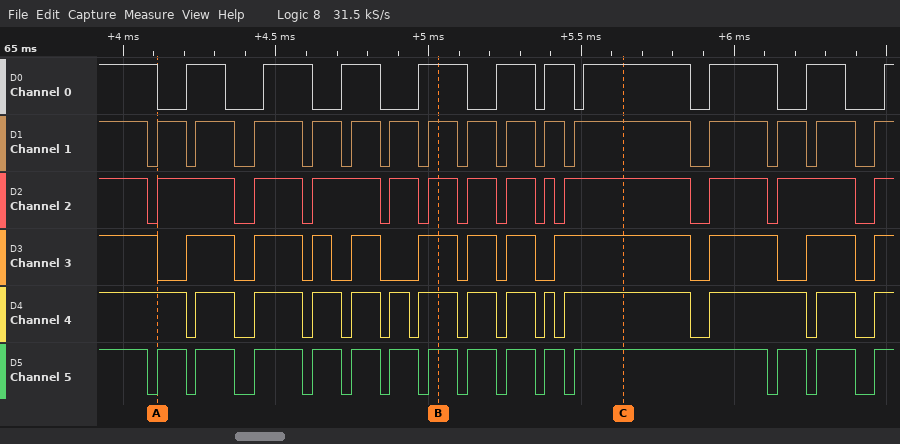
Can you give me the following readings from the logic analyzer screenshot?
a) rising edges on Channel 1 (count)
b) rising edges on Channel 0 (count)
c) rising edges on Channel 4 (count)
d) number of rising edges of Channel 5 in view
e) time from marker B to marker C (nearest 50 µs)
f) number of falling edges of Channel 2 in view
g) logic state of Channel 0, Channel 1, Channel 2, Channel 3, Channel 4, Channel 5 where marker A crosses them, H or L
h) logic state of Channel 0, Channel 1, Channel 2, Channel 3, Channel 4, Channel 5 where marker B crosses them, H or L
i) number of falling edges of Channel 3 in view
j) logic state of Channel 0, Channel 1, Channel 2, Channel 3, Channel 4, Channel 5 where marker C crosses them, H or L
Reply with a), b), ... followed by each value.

a) 15
b) 10
c) 13
d) 14
e) 600 µs
f) 12
g) Channel 0=L, Channel 1=H, Channel 2=H, Channel 3=L, Channel 4=H, Channel 5=H
h) Channel 0=H, Channel 1=H, Channel 2=H, Channel 3=H, Channel 4=H, Channel 5=H
i) 11
j) Channel 0=H, Channel 1=H, Channel 2=H, Channel 3=H, Channel 4=H, Channel 5=H
